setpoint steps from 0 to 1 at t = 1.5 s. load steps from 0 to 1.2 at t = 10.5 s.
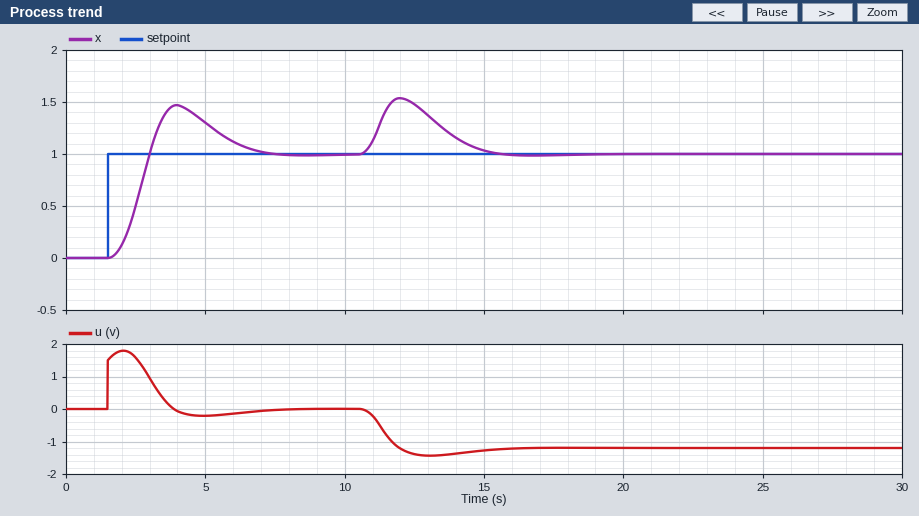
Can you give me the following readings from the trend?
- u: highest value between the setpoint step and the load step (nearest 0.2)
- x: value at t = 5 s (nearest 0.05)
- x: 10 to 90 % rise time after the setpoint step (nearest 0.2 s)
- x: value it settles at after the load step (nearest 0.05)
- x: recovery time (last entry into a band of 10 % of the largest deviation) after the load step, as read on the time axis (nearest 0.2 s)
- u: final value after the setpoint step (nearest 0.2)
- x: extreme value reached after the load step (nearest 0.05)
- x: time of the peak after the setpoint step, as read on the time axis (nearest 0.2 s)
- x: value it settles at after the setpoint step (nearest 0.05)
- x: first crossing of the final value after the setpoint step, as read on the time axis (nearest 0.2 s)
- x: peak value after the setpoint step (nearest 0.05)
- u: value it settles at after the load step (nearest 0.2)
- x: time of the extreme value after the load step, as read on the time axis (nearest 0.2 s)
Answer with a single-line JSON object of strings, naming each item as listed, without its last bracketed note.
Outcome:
{"u: highest value between the setpoint step and the load step": "1.8", "x: value at t = 5 s": "1.30", "x: 10 to 90 % rise time after the setpoint step": "1.0 s", "x: value it settles at after the load step": "1.00", "x: recovery time (last entry into a band of 10 % of the largest deviation) after the load step, as read on the time axis": "14.8 s", "u: final value after the setpoint step": "0.0", "x: extreme value reached after the load step": "1.55", "x: time of the peak after the setpoint step, as read on the time axis": "4.0 s", "x: value it settles at after the setpoint step": "1.00", "x: first crossing of the final value after the setpoint step, as read on the time axis": "3.0 s", "x: peak value after the setpoint step": "1.45", "u: value it settles at after the load step": "-1.2", "x: time of the extreme value after the load step, as read on the time axis": "12.0 s"}
